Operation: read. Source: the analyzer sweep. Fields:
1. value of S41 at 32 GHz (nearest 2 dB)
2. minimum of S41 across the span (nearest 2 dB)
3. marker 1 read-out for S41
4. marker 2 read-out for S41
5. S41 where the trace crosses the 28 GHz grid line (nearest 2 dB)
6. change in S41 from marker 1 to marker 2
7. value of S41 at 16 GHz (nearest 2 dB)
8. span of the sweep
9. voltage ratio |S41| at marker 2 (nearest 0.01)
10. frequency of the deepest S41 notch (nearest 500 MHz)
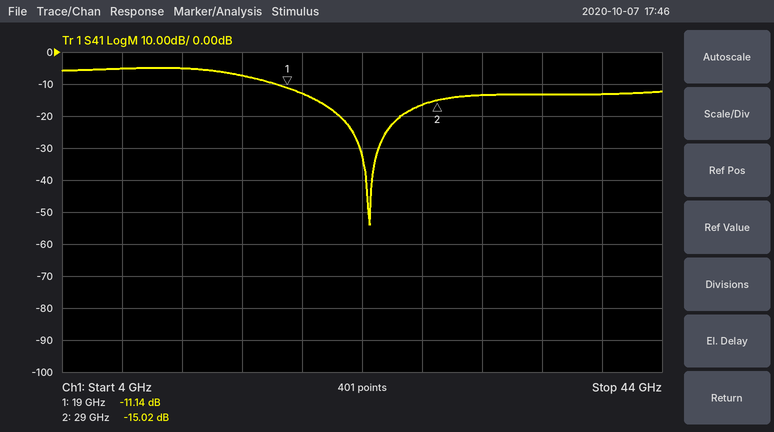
-14 dB
-54 dB
-11.14 dB
-15.02 dB
-16 dB
-3.88 dB
-8 dB
40 GHz
0.18
24.5 GHz
